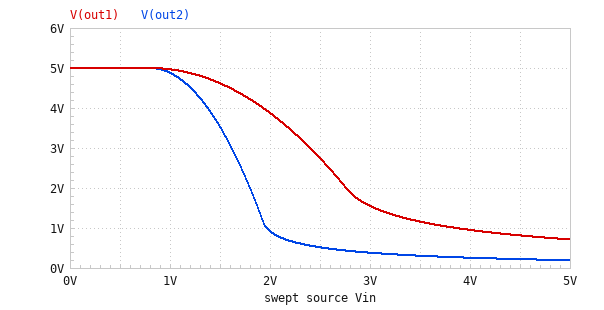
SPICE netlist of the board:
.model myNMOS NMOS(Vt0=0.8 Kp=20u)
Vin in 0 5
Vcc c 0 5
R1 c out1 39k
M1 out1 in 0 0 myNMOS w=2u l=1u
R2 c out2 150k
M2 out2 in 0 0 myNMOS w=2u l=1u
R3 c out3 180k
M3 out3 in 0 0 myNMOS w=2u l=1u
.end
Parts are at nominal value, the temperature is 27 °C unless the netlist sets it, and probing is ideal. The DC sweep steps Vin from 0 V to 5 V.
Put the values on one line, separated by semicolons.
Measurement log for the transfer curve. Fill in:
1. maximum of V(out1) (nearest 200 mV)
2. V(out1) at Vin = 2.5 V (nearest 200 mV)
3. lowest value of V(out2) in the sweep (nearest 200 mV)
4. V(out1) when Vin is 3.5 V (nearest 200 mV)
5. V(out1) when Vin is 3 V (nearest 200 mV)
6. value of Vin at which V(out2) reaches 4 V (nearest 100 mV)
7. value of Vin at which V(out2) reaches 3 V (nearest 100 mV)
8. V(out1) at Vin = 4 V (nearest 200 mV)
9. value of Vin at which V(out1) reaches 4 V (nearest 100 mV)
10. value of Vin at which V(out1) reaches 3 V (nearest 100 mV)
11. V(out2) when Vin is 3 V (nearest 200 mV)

5.0 V; 2.8 V; 200 mV; 1.2 V; 1.6 V; 1.4 V; 1.6 V; 1.0 V; 1.9 V; 2.4 V; 400 mV
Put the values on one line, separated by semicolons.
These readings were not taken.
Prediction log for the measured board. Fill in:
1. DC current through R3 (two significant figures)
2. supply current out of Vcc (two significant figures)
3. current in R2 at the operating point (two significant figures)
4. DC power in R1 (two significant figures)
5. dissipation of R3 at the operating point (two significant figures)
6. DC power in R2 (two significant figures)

27 µA; 170 µA; 32 µA; 470 µW; 130 µW; 150 µW
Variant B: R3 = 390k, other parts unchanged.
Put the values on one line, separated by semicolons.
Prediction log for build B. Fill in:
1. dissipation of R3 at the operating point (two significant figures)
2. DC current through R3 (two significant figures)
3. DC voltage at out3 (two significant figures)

62 µW; 13 µA; 76 mV
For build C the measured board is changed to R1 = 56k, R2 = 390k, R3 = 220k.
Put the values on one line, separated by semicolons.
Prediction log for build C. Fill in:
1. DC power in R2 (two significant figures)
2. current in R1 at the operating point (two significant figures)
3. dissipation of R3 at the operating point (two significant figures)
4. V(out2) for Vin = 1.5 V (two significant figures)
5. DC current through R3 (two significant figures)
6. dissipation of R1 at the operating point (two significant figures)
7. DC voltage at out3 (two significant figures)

62 µW; 80 µA; 110 µW; 1.2 V; 22 µA; 360 µW; 130 mV
